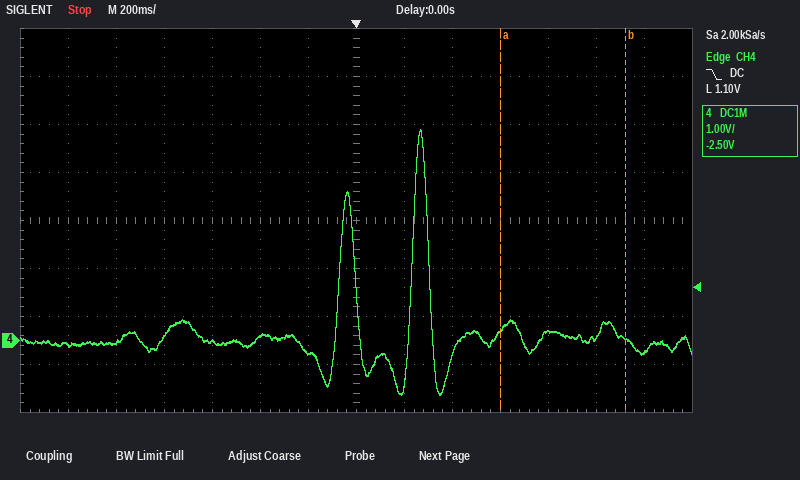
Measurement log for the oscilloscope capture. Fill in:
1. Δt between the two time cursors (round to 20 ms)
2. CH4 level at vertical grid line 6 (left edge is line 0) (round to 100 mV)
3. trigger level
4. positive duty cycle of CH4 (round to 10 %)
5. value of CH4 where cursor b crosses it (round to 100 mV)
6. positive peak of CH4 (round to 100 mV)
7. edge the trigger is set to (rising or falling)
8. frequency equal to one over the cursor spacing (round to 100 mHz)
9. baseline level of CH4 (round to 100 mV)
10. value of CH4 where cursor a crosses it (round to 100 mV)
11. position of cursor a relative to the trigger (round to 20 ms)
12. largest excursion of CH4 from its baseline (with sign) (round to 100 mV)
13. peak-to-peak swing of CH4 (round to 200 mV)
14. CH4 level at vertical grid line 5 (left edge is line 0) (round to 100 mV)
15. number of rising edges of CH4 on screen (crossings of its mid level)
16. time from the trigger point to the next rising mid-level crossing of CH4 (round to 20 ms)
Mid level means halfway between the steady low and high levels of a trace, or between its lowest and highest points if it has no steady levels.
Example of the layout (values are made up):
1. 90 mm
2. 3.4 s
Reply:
1. 520 ms
2. -300 mV
3. 1.10 V
4. 20 %
5. 0.0 V
6. 4.4 V
7. falling
8. 1.9 Hz
9. 0.0 V
10. 200 mV
11. +600 ms
12. +4.4 V
13. 5.6 V
14. 100 mV
15. 2
16. 240 ms
